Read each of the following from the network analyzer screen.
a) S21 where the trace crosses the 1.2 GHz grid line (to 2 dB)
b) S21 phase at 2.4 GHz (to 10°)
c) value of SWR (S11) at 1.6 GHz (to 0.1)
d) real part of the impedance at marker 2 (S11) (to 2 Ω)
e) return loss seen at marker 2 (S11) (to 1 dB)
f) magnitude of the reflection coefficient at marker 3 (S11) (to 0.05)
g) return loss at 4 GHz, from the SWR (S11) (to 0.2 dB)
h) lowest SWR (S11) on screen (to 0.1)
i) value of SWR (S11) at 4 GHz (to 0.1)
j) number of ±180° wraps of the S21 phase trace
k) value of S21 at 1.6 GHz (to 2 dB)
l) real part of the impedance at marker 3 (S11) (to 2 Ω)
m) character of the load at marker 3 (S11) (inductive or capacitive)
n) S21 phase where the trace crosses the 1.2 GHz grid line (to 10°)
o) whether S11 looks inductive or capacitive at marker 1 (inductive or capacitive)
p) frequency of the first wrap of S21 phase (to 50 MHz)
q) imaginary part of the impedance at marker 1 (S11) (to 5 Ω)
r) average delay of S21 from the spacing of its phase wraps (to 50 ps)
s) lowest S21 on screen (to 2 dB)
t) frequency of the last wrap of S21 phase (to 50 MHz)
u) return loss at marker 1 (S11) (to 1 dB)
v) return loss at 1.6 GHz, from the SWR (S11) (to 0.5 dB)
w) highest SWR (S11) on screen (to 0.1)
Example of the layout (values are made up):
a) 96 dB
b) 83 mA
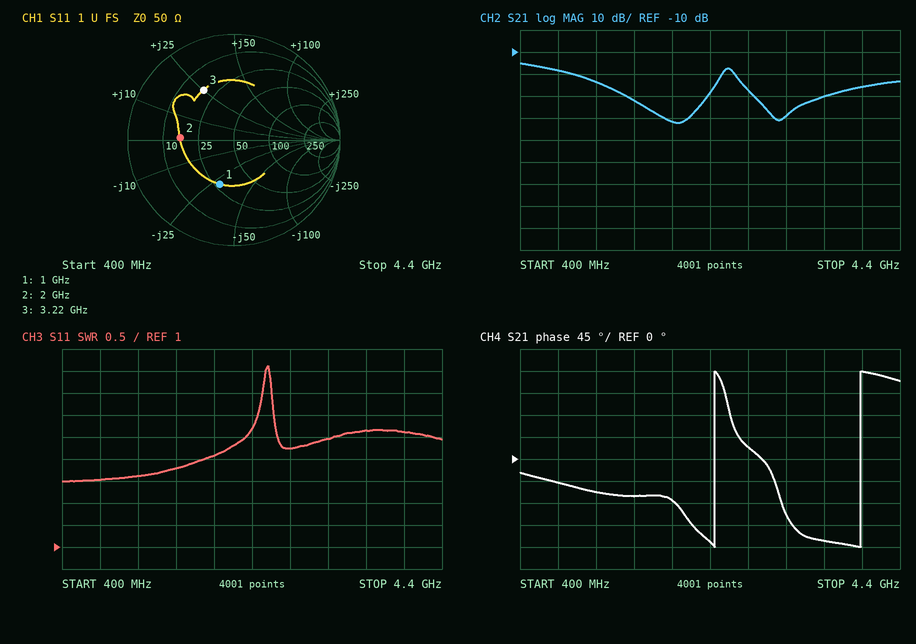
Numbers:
a) -24 dB
b) -170°
c) 2.8
d) 16 Ω
e) 6 dB
f) 0.55
g) 5.0 dB
h) 2.5
i) 3.6
j) 2
k) -32 dB
l) 18 Ω
m) inductive
n) -70°
o) capacitive
p) 2.45 GHz
q) -30 Ω
r) 650 ps
s) -42 dB
t) 4.00 GHz
u) 7 dB
v) 6.5 dB
w) 5.1
